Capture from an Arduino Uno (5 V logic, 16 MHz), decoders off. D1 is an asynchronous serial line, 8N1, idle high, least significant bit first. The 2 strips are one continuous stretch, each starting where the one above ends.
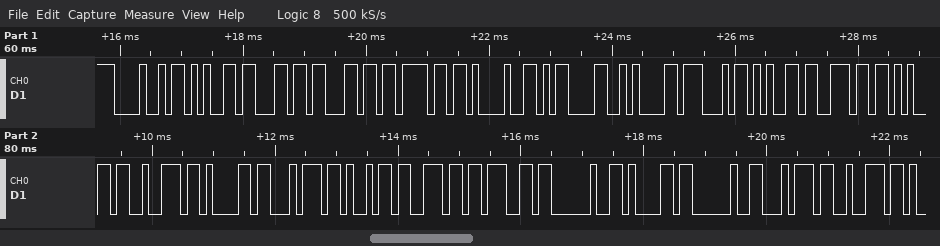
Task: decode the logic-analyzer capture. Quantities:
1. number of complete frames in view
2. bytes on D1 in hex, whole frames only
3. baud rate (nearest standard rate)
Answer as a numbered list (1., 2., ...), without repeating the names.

1. 23
2. 48 65 6C 6C 6F 21 0D 0A 47 65 6E 65 72 61 74 69 6E 67 20 61 20 74 72
3. 9600 baud
